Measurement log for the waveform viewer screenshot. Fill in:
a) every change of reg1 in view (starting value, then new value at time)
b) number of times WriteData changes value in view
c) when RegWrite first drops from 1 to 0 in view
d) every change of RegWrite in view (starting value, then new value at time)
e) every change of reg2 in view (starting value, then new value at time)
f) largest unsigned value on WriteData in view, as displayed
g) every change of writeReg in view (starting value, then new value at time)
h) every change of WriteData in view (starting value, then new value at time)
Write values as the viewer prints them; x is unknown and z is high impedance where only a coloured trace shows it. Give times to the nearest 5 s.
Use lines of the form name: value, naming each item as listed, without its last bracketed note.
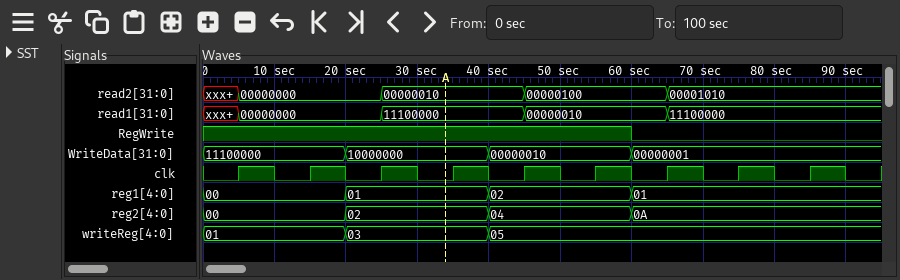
every change of reg1 in view: 00, 01 at 20 s, 02 at 40 s, 01 at 60 s
number of times WriteData changes value in view: 3
when RegWrite first drops from 1 to 0 in view: 60 s
every change of RegWrite in view: 1, 0 at 60 s
every change of reg2 in view: 00, 02 at 20 s, 04 at 40 s, 0A at 60 s
largest unsigned value on WriteData in view, as displayed: 11100000
every change of writeReg in view: 01, 03 at 20 s, 05 at 40 s
every change of WriteData in view: 11100000, 10000000 at 20 s, 00000010 at 40 s, 00000001 at 60 s
